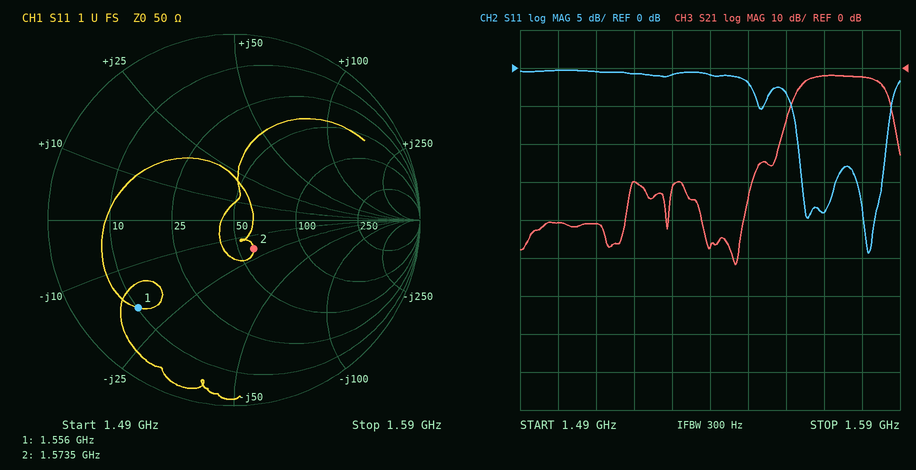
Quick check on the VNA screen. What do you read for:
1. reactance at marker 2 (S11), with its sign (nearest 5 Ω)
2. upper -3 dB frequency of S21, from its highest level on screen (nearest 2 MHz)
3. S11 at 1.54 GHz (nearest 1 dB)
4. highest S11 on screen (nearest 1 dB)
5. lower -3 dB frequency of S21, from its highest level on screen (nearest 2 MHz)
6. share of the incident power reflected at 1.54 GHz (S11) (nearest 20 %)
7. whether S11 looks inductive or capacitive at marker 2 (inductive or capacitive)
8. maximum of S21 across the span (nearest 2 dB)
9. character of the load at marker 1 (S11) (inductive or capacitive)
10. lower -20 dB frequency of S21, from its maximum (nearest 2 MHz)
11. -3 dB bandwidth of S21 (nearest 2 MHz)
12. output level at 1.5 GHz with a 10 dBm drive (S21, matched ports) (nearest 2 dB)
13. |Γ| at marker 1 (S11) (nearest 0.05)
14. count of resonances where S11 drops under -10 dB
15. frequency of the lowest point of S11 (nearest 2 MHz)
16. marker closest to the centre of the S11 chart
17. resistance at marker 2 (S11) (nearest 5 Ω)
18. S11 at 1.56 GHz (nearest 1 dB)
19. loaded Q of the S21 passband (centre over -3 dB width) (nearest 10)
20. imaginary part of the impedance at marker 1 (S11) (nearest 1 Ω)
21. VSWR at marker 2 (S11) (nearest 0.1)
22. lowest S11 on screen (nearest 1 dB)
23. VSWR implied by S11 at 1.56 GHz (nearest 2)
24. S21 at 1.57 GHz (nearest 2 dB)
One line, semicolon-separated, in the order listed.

-20 Ω; 1.586 GHz; -1 dB; 0 dB; 1.564 GHz; 80 %; capacitive; -2 dB; capacitive; 1.558 GHz; 22 MHz; -30 dBm; 0.70; 2; 1.582 GHz; marker 2; 60 Ω; -3 dB; 70; -19 Ω; 1.5; -24 dB; 6; -2 dB
